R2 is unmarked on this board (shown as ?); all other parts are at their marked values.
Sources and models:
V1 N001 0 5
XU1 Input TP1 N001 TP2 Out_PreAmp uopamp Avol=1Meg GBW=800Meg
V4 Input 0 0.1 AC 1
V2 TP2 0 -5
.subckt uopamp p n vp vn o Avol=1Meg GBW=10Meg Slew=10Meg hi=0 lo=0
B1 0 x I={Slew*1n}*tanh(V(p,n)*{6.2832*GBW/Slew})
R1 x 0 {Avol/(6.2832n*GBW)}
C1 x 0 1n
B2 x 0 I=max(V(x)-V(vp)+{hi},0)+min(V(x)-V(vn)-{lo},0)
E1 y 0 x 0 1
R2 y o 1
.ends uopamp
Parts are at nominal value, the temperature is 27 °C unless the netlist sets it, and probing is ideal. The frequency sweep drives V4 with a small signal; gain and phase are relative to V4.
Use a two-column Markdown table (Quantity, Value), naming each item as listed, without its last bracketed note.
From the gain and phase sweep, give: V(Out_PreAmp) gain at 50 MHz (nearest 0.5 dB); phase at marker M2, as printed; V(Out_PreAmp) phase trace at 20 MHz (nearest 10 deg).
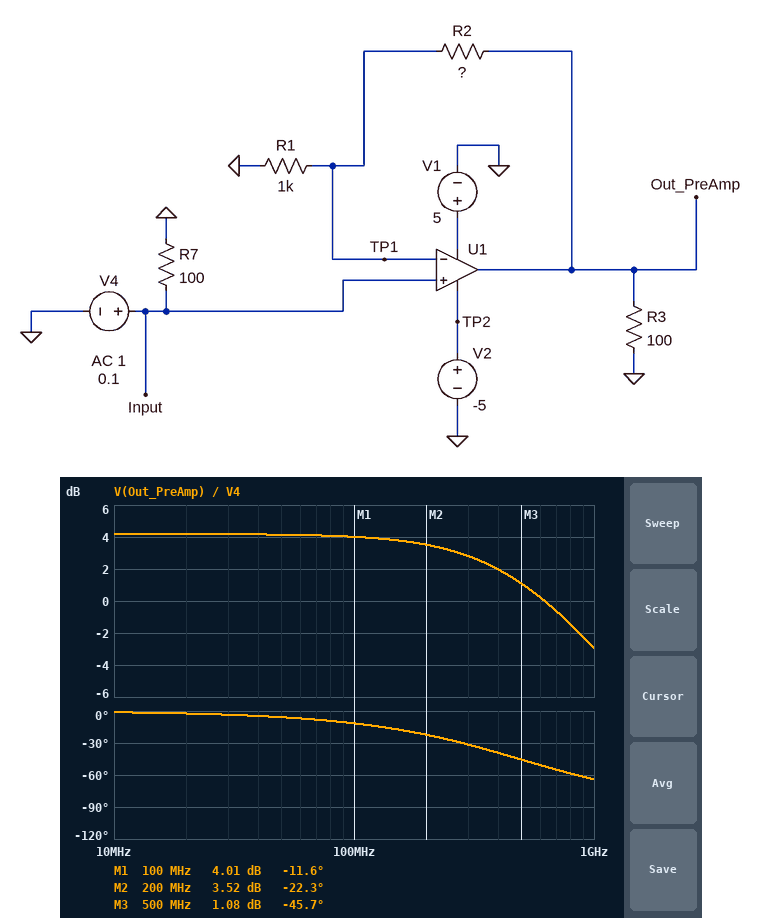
| Quantity | Value |
|---|---|
| V(Out_PreAmp) gain at 50 MHz | 4.0 dB |
| phase at marker M2, as printed | -22.3 deg |
| V(Out_PreAmp) phase trace at 20 MHz | 0 deg |
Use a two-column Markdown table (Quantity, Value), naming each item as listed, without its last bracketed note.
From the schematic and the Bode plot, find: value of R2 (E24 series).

| Quantity | Value |
|---|---|
| value of R2 | 620 Ω |
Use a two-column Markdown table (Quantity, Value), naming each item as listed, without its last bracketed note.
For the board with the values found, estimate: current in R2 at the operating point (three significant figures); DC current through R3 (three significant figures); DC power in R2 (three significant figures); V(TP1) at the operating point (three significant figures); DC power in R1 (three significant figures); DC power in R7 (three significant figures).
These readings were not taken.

| Quantity | Value |
|---|---|
| current in R2 at the operating point | 100 µA |
| DC current through R3 | 1.62 mA |
| DC power in R2 | 6.20 µW |
| V(TP1) at the operating point | 100 mV |
| DC power in R1 | 10.0 µW |
| DC power in R7 | 100 µW |
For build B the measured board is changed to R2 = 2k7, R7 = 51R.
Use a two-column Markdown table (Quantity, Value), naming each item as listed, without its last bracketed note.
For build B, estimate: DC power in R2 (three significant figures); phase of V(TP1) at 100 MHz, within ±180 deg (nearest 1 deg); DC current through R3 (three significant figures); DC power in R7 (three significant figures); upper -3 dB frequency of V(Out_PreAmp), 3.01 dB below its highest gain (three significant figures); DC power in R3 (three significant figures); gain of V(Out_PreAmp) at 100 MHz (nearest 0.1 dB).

| Quantity | Value |
|---|---|
| DC power in R2 | 27.0 µW |
| phase of V(TP1) at 100 MHz, within ±180 deg | -25 deg |
| DC current through R3 | 3.70 mA |
| DC power in R7 | 196 µW |
| upper -3 dB frequency of V(Out_PreAmp), 3.01 dB below its highest gain | 214 MHz |
| DC power in R3 | 1.37 mW |
| gain of V(Out_PreAmp) at 100 MHz | 10.5 dB |
